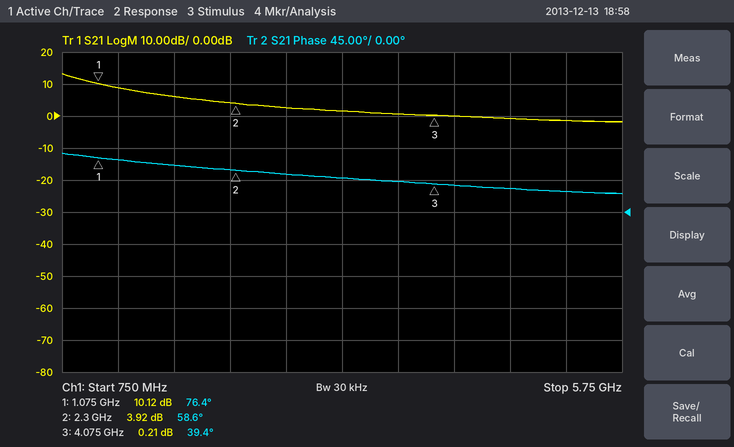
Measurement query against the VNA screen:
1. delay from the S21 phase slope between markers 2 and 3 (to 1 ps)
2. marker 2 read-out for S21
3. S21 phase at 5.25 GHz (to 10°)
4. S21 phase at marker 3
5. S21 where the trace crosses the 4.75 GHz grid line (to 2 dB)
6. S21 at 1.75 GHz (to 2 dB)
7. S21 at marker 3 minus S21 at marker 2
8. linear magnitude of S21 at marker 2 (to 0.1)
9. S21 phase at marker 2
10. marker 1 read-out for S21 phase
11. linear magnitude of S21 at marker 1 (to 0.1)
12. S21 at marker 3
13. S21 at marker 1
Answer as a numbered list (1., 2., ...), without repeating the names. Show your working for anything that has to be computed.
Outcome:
1. −(39.4° − (58.6°))/(360° × 1.775 GHz) ≈ 30 ps
2. 3.92 dB
3. 30°
4. 39.4°
5. 0 dB
6. 6 dB
7. 0.21 − (3.92) = -3.71 dB
8. 10^(3.92/20) ≈ 1.6
9. 58.6°
10. 76.4°
11. 10^(10.12/20) ≈ 3.2
12. 0.21 dB
13. 10.12 dB
